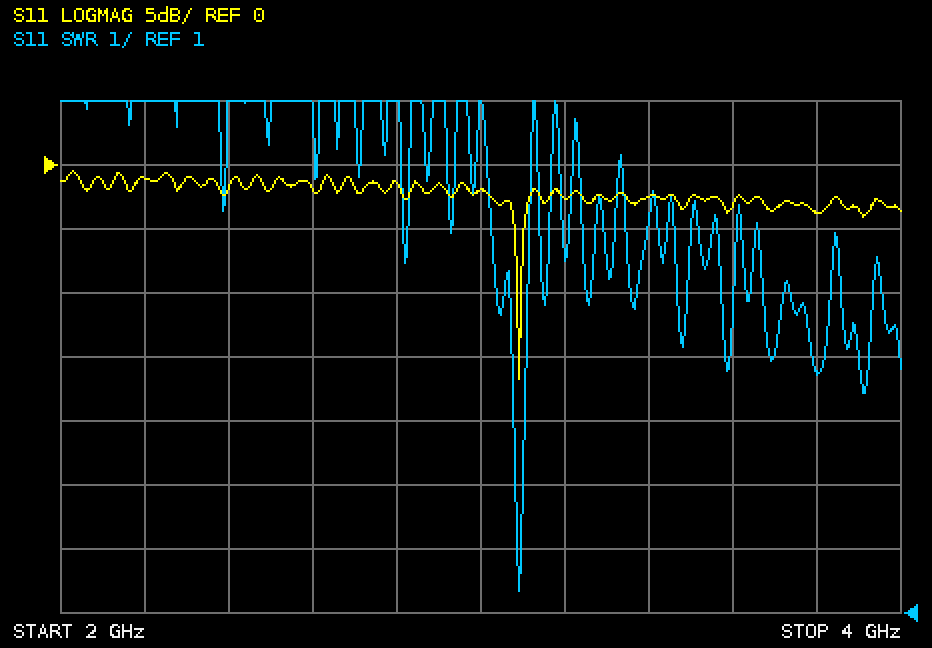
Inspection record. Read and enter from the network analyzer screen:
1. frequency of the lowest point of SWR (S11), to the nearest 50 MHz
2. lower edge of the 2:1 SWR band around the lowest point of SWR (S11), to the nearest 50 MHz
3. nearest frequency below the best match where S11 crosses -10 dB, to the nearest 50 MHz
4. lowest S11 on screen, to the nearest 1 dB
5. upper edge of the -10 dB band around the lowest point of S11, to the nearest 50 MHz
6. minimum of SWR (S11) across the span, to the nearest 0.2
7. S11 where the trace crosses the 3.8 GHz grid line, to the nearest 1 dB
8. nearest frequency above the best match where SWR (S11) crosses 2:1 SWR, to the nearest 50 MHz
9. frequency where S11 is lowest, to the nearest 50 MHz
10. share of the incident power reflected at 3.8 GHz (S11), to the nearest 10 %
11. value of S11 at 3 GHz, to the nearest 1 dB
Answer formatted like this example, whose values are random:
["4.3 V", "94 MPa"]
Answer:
["3.10 GHz", "3.10 GHz", "3.10 GHz", "-17 dB", "3.10 GHz", "1.4", "-4 dB", "3.10 GHz", "3.10 GHz", "40 %", "-2 dB"]
